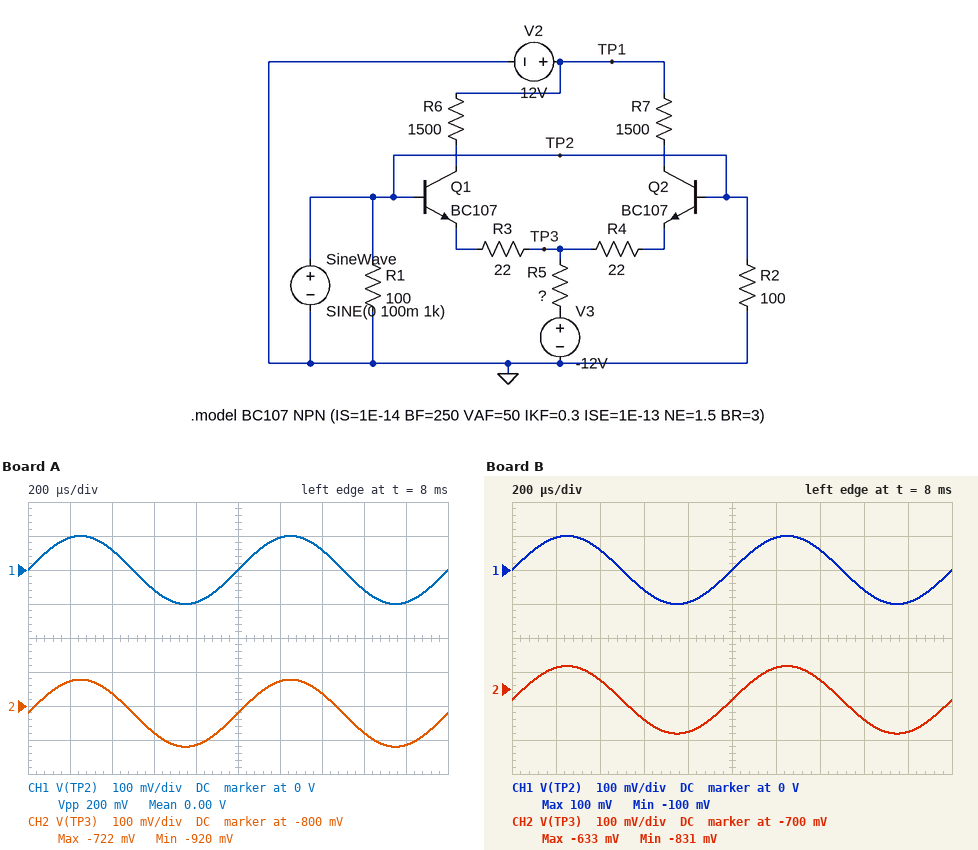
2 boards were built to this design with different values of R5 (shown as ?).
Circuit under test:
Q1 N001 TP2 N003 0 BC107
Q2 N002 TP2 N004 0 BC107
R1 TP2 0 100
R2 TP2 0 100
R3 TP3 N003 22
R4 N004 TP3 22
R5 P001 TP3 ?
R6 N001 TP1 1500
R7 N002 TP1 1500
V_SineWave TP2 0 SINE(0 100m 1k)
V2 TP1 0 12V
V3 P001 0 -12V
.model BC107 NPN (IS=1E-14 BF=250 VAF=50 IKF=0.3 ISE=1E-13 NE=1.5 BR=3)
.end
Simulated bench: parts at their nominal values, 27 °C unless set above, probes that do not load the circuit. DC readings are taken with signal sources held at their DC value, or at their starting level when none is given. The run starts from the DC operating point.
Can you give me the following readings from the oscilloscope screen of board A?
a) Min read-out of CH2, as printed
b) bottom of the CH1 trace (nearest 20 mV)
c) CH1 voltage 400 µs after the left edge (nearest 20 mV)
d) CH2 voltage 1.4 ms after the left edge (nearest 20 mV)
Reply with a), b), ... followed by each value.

a) -920 mV
b) -100 mV
c) 60 mV
d) -760 mV
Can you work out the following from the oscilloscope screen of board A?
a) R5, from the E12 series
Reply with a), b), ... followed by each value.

a) 1 kΩ
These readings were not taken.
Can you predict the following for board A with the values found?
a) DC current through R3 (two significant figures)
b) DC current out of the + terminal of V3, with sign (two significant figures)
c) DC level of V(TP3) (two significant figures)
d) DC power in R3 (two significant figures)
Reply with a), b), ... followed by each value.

a) 5.6 mA
b) -11 mA
c) -820 mV
d) 690 µW
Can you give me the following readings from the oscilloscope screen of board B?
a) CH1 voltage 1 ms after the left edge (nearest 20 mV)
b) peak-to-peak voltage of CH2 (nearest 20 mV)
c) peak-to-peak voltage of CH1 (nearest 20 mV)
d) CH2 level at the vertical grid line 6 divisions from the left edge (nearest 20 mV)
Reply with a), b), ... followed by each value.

a) 0 V
b) 200 mV
c) 200 mV
d) -640 mV
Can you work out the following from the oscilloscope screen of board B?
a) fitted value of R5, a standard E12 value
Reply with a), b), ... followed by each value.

a) 2.2 kΩ
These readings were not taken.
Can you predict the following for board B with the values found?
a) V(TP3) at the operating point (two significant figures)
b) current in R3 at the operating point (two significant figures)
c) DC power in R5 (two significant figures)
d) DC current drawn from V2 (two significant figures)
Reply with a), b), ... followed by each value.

a) -730 mV
b) 2.6 mA
c) 58 mW
d) 5.1 mA
